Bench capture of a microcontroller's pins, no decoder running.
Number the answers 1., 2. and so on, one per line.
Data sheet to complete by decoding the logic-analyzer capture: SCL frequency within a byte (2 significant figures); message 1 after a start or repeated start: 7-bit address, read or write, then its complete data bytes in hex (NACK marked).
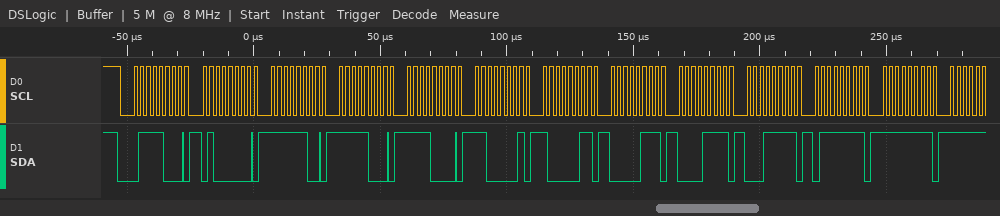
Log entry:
1. 400 kHz
2. 0x3C write: 40 FC F8 F0 C1 83 07 0F 1F 7F FF
